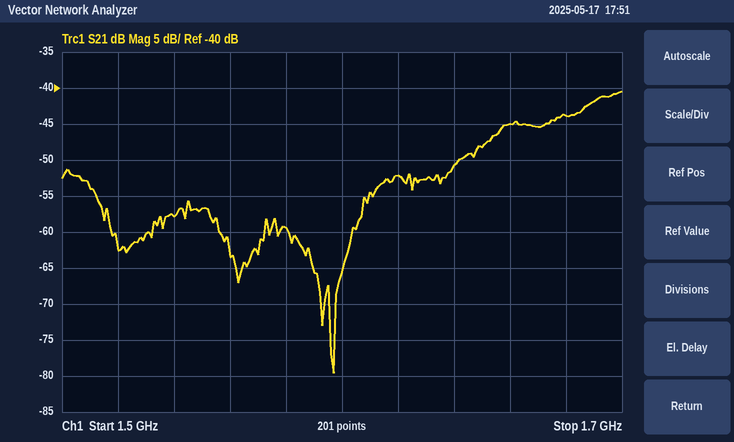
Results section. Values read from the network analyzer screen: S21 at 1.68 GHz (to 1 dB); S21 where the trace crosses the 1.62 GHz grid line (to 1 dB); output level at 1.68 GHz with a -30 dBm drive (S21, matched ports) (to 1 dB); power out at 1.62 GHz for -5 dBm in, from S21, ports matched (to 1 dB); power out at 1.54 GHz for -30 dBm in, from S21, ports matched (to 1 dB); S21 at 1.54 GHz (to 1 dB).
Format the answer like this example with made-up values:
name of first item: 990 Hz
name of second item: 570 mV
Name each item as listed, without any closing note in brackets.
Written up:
S21 at 1.68 GHz: -44 dB
S21 where the trace crosses the 1.62 GHz grid line: -52 dB
output level at 1.68 GHz with a -30 dBm drive (S21, matched ports): -74 dBm
power out at 1.62 GHz for -5 dBm in, from S21, ports matched: -57 dBm
power out at 1.54 GHz for -30 dBm in, from S21, ports matched: -88 dBm
S21 at 1.54 GHz: -58 dB
